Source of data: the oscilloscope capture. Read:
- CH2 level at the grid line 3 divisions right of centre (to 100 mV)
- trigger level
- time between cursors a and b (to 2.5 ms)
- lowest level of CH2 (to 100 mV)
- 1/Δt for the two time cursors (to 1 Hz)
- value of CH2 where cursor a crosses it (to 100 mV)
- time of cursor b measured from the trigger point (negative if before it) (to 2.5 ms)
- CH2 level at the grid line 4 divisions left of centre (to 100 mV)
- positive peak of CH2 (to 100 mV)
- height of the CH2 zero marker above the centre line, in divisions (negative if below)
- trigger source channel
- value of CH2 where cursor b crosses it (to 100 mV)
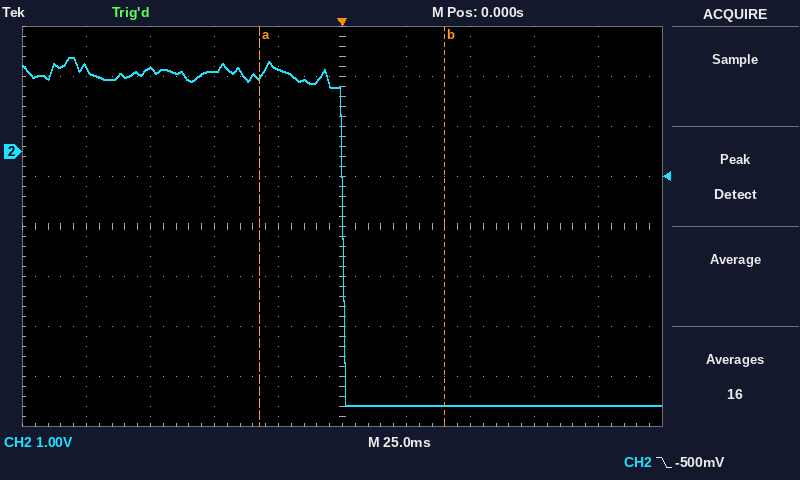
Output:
-5.1 V
-500 mV
72.5 ms
-5.1 V
14 Hz
1.5 V
+40.0 ms
1.7 V
1.9 V
+1.5 div
CH2
-5.1 V
